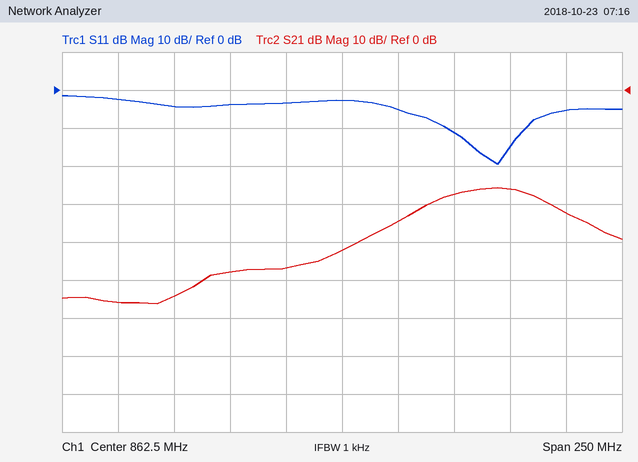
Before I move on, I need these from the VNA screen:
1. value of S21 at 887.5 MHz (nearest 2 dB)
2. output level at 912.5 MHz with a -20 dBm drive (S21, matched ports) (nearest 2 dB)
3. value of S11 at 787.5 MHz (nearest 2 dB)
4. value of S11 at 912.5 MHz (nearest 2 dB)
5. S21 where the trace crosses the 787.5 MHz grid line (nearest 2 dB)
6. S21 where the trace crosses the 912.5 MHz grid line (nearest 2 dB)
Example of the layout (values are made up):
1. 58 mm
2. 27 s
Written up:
1. -34 dB
2. -48 dBm
3. -4 dB
4. -12 dB
5. -54 dB
6. -28 dB
